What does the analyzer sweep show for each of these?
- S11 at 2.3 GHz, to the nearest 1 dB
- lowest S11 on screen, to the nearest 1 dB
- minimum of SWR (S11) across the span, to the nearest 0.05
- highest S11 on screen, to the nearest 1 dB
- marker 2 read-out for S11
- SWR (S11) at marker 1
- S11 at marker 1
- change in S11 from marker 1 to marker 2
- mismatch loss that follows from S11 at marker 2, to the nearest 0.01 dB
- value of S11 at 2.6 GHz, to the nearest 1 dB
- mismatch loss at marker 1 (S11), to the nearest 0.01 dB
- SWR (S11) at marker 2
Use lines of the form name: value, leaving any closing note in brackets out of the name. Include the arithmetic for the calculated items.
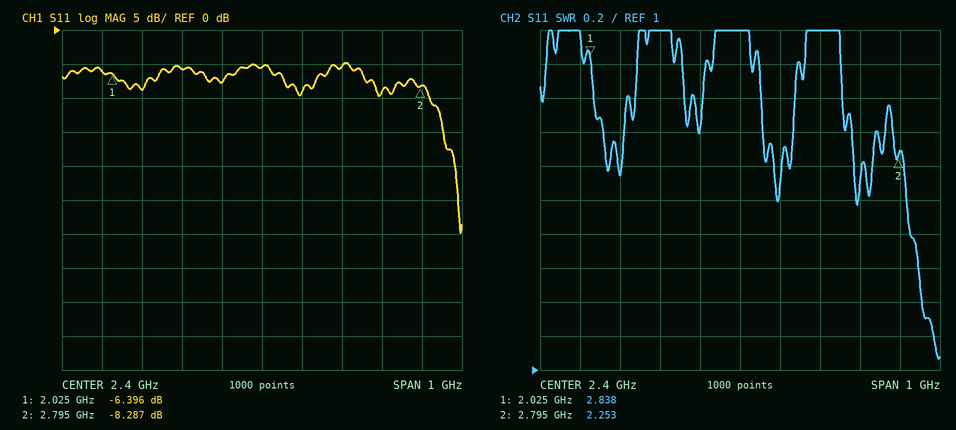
S11 at 2.3 GHz, to the nearest 1 dB: -8 dB
lowest S11 on screen, to the nearest 1 dB: -30 dB
minimum of SWR (S11) across the span, to the nearest 0.05: 1.05
highest S11 on screen, to the nearest 1 dB: -5 dB
marker 2 read-out for S11: -8.287 dB
SWR (S11) at marker 1: 2.838
S11 at marker 1: -6.396 dB
change in S11 from marker 1 to marker 2: -8.287 − (-6.396) = -1.891 dB
mismatch loss that follows from S11 at marker 2, to the nearest 0.01 dB: −10 log10(1 − 10^(-8.287/10)) ≈ 0.70 dB
value of S11 at 2.6 GHz, to the nearest 1 dB: -5 dB
mismatch loss at marker 1 (S11), to the nearest 0.01 dB: −10 log10(1 − 10^(-6.396/10)) ≈ 1.13 dB
SWR (S11) at marker 2: 2.253
